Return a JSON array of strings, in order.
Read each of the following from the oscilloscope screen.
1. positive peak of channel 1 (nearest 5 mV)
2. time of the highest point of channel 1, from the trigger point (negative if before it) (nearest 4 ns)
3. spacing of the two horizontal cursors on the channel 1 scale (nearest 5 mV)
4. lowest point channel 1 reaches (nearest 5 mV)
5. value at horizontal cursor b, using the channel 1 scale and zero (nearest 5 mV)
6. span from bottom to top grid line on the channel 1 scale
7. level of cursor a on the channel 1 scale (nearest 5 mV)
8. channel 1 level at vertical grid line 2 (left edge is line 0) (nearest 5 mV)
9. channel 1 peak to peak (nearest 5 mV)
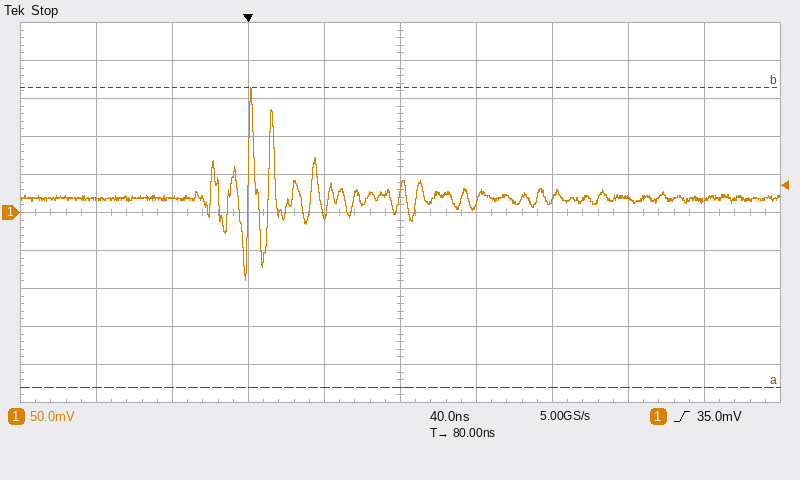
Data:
["165 mV", "0 ns", "395 mV", "-90 mV", "165 mV", "500 mV", "-230 mV", "20 mV", "255 mV"]
